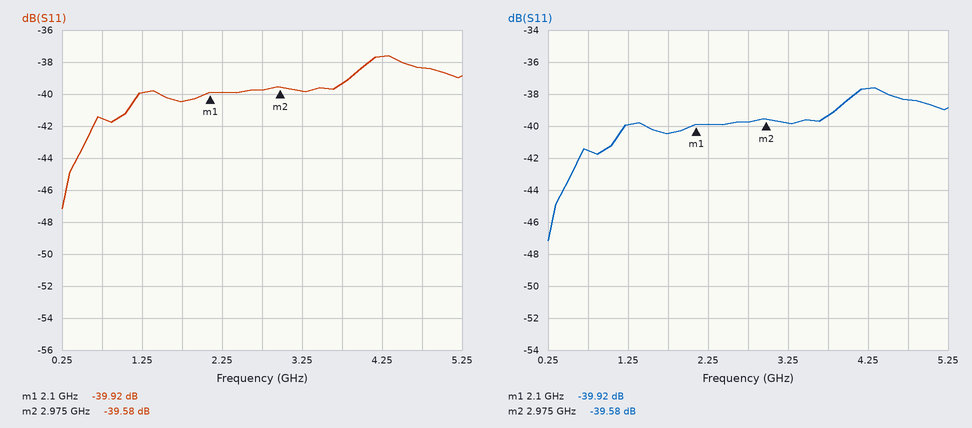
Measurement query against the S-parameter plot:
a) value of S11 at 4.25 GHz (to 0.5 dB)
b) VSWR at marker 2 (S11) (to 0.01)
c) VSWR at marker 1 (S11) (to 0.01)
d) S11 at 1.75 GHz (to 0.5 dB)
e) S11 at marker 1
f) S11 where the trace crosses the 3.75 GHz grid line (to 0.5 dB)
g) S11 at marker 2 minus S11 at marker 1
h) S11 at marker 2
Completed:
-37.5 dB
1.02
1.02
-40.5 dB
-39.92 dB
-39.5 dB
0.34 dB
-39.58 dB
